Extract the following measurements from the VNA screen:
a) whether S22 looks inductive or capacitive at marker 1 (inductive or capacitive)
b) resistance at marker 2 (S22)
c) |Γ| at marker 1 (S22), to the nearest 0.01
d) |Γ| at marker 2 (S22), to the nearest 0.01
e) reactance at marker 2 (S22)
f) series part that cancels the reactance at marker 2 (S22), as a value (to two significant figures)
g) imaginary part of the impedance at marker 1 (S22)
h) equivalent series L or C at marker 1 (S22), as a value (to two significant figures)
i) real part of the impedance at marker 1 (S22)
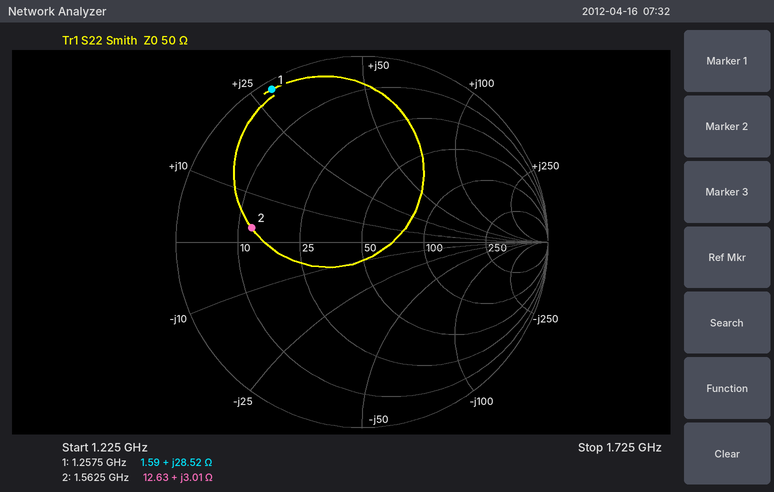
inductive
12.63 Ω
0.95
0.60
+3.01 Ω
34 pF
+28.52 Ω
3.6 nH
1.59 Ω
